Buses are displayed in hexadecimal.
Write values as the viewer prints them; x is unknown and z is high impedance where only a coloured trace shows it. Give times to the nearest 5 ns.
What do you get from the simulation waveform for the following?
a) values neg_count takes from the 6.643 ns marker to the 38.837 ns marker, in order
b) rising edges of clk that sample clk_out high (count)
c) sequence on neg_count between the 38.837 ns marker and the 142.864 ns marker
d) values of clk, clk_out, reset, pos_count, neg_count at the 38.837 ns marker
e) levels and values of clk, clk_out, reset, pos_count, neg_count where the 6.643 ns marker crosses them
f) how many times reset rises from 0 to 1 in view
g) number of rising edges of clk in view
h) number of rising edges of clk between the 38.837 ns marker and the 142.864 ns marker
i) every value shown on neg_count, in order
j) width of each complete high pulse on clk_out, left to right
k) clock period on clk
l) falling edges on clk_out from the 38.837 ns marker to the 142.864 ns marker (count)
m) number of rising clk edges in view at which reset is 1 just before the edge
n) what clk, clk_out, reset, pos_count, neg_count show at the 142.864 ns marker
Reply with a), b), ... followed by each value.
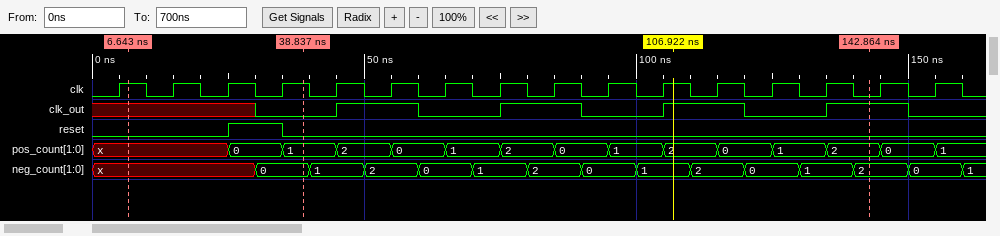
a) x, 0
b) 4
c) 0, 1, 2, 0, 1, 2, 0, 1, 2, 0, 1, 2
d) clk=1, clk_out=0, reset=0, pos_count=1, neg_count=0
e) clk=1, clk_out=x, reset=0, pos_count=x, neg_count=x
f) 1
g) 16
h) 10
i) x, 0, 1, 2, 0, 1, 2, 0, 1, 2, 0, 1, 2, 0, 1
j) 15 ns, 15 ns, 15 ns, 15 ns
k) 10 ns
l) 3
m) 1
n) clk=0, clk_out=1, reset=0, pos_count=2, neg_count=2
